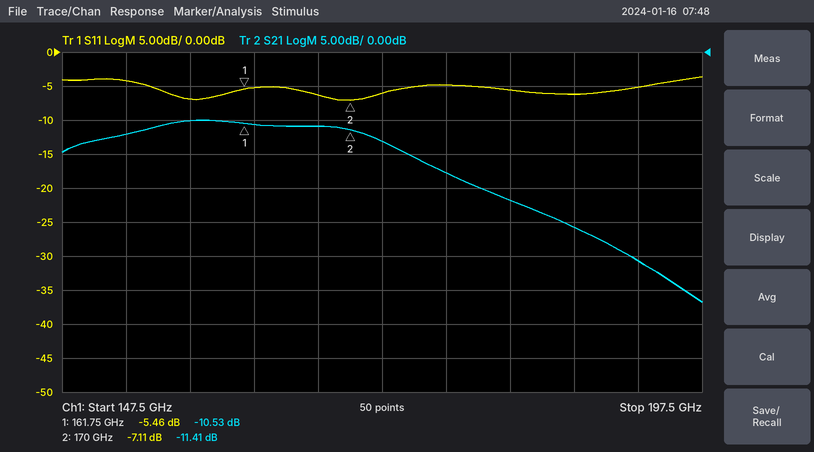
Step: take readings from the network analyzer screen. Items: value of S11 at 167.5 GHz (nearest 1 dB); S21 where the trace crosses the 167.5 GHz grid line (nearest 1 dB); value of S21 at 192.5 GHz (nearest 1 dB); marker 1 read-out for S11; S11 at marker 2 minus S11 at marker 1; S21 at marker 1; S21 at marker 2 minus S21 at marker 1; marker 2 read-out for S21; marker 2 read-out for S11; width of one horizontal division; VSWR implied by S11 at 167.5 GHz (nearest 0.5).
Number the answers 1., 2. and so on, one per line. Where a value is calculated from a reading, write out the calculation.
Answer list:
1. -6 dB
2. -11 dB
3. -31 dB
4. -5.46 dB
5. -7.11 − (-5.46) = -1.65 dB
6. -10.53 dB
7. -11.41 − (-10.53) = -0.88 dB
8. -11.41 dB
9. -7.11 dB
10. 5 GHz
11. |Γ| = 10^(-6/20) = 0.5012; VSWR = (1 + 0.5012)/(1 − 0.5012) ≈ 3.0
